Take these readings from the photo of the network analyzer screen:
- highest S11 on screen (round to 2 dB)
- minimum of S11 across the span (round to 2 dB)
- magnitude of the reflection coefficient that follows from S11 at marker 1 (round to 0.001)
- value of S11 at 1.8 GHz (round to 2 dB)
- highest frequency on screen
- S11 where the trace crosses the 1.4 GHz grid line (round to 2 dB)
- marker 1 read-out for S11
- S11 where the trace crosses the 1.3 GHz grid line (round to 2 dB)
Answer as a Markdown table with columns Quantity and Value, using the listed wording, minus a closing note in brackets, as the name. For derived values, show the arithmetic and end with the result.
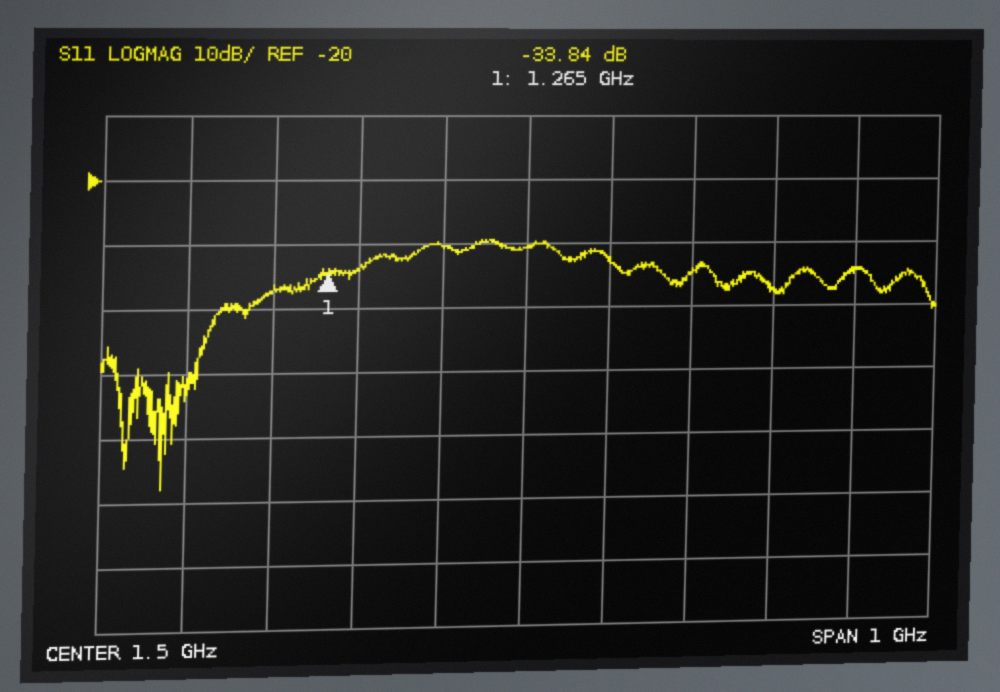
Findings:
| Quantity | Value |
|---|---|
| highest S11 on screen | -30 dB |
| minimum of S11 across the span | -68 dB |
| magnitude of the reflection coefficient that follows from S11 at marker 1 | 10^(-33.84/20) ≈ 0.020 |
| value of S11 at 1.8 GHz | -38 dB |
| highest frequency on screen | 2 GHz |
| S11 where the trace crosses the 1.4 GHz grid line | -30 dB |
| marker 1 read-out for S11 | -33.84 dB |
| S11 where the trace crosses the 1.3 GHz grid line | -34 dB |
